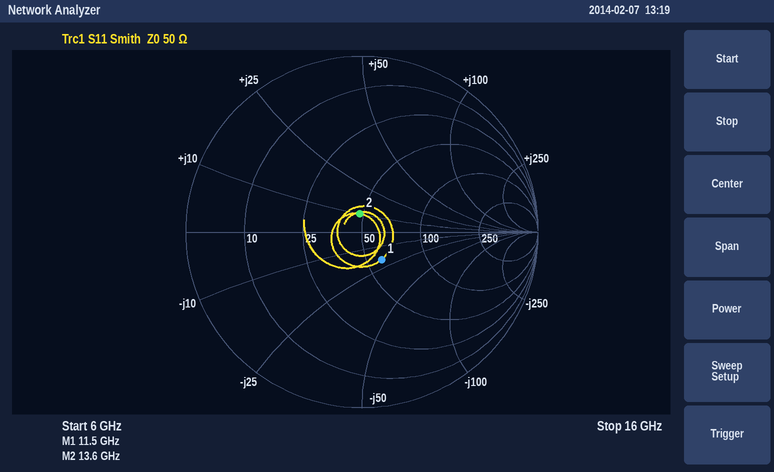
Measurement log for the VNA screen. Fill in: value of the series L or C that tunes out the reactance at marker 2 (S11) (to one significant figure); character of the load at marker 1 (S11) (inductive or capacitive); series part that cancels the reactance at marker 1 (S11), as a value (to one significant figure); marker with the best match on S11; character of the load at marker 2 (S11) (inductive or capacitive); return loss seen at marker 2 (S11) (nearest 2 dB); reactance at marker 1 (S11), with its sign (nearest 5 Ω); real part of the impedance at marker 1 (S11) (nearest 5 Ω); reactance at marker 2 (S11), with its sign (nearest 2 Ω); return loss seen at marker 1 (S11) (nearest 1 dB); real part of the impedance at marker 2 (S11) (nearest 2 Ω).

1 pF
capacitive
300 pH
marker 2
inductive
20 dB
-20 Ω
60 Ω
+10 Ω
14 dB
48 Ω
